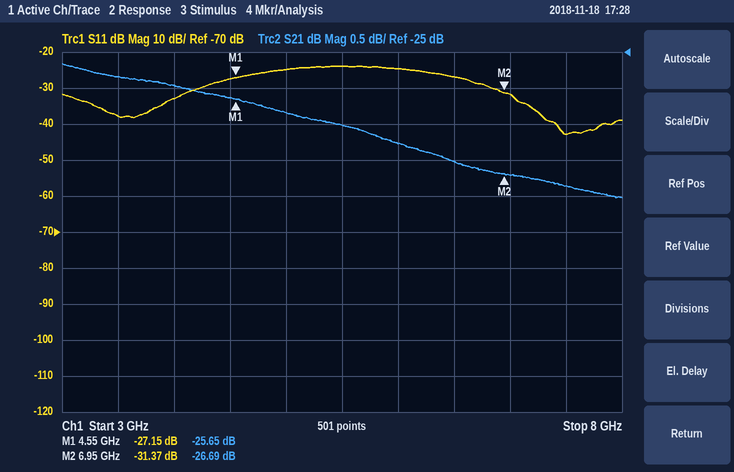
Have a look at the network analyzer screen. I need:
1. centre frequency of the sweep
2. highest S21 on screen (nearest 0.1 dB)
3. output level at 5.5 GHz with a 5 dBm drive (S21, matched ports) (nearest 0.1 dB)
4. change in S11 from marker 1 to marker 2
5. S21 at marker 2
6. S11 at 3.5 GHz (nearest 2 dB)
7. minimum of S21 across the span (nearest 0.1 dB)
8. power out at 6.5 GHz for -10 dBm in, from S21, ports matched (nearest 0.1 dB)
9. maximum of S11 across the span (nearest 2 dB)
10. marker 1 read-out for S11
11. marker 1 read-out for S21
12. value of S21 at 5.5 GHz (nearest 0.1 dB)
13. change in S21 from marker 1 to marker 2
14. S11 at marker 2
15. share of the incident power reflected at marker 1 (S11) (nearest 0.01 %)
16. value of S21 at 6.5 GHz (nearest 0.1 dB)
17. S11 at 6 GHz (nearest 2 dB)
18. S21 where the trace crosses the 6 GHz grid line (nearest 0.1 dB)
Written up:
5.5 GHz
-25.2 dB
-21.0 dBm
-4.22 dB
-26.69 dB
-38 dB
-27.0 dB
-36.5 dBm
-24 dB
-27.15 dB
-25.65 dB
-26.0 dB
-1.04 dB
-31.37 dB
0.19 %
-26.5 dB
-24 dB
-26.3 dB
